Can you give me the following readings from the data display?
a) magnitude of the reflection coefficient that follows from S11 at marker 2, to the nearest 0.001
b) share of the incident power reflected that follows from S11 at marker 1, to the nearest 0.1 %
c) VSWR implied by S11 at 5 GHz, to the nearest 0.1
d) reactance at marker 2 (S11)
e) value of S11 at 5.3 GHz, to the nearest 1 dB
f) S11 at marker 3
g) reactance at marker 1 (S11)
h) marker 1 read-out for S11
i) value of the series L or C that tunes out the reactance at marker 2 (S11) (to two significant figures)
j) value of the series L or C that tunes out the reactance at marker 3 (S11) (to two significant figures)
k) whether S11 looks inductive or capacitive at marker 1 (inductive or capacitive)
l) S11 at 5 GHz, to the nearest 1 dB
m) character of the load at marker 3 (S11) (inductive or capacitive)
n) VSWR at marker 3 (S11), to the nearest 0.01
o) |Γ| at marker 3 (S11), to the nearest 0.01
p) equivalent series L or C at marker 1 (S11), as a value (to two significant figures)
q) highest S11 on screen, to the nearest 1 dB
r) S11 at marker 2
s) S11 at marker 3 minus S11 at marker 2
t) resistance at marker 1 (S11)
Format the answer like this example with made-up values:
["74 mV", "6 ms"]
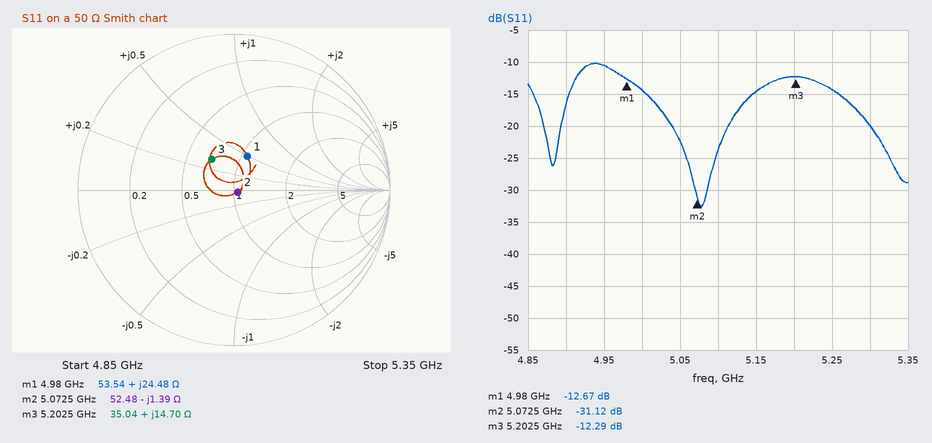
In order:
["0.028", "5.4 %", "1.5", "-1.39 Ω", "-20 dB", "-12.29 dB", "+24.48 Ω", "-12.67 dB", "44 pH", "2.1 pF", "inductive", "-14 dB", "inductive", "1.64", "0.24", "780 pH", "-10 dB", "-31.12 dB", "18.83 dB", "53.54 Ω"]
